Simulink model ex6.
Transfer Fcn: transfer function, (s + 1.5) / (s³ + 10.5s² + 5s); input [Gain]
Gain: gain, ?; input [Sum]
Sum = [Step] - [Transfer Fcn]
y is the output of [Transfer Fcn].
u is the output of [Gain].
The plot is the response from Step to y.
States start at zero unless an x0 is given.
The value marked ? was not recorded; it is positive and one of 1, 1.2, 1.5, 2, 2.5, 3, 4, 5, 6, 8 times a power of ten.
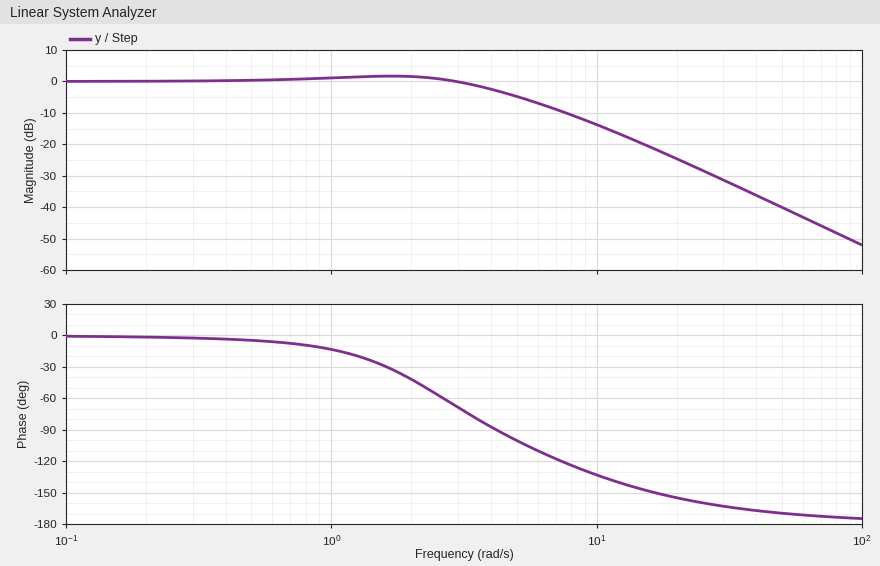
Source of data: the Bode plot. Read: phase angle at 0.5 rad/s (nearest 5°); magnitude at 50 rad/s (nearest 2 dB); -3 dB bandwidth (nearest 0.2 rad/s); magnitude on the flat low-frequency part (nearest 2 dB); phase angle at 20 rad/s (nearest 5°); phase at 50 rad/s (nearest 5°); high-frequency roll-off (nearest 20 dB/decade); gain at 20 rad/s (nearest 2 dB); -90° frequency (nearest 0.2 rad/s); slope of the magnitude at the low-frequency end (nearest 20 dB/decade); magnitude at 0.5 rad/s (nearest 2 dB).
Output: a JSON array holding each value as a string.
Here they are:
["-5°", "-40 dB", "4.2 rad/s", "0 dB", "-155°", "-170°", "-40 dB/decade", "-24 dB", "4.2 rad/s", "0 dB/decade", "0 dB"]
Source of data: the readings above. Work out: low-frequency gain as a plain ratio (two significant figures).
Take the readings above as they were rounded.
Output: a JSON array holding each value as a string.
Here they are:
["1.0"]
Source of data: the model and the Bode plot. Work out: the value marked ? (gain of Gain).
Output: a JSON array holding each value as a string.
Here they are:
["25"]
